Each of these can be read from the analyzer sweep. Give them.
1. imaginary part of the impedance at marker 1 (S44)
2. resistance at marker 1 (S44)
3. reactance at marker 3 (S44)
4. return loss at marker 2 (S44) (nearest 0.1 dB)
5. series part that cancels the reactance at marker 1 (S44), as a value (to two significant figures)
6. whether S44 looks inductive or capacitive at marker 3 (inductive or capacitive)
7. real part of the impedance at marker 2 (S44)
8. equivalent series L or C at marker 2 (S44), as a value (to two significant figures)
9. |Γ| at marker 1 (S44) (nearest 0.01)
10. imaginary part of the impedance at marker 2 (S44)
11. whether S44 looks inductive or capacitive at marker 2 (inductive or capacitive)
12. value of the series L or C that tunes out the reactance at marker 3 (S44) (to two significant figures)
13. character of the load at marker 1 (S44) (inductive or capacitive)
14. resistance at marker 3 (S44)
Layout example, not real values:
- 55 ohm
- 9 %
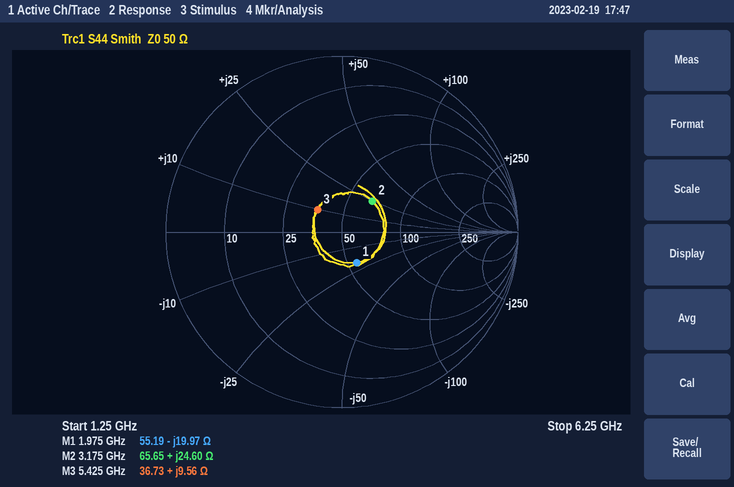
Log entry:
- -19.97 Ω
- 55.19 Ω
- +9.56 Ω
- 12.2 dB
- 1.6 nH
- inductive
- 65.65 Ω
- 1.2 nH
- 0.19
- +24.60 Ω
- inductive
- 3.1 pF
- capacitive
- 36.73 Ω
